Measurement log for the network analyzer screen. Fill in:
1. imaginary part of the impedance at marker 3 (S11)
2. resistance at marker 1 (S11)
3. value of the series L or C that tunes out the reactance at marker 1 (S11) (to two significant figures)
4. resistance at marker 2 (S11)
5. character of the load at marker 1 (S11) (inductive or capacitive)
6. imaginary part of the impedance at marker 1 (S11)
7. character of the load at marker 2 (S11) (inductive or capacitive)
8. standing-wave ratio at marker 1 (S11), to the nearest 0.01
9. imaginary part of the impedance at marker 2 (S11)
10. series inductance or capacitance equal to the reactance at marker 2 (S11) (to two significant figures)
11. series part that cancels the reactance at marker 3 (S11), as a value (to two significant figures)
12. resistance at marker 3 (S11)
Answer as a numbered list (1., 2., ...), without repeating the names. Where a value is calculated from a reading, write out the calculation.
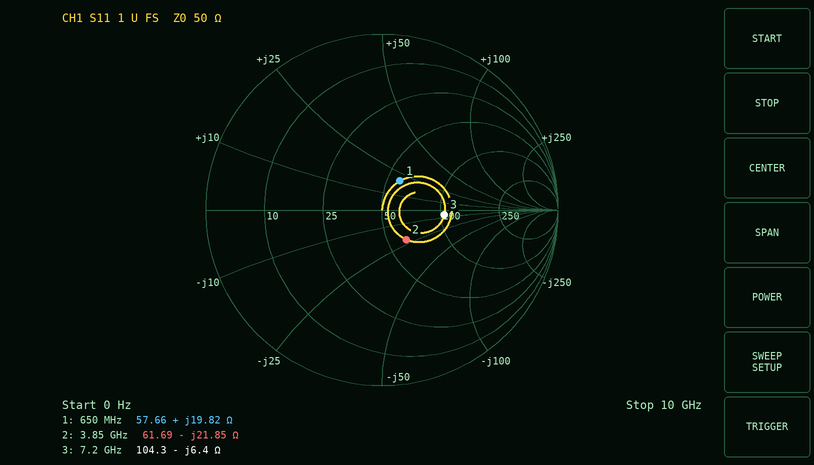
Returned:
1. -6.4 Ω
2. 57.66 Ω
3. C = 1/(2π × 650 MHz × 19.82 Ω) ≈ 12 pF
4. 61.69 Ω
5. inductive
6. +19.82 Ω
7. capacitive
8. 1.48
9. -21.85 Ω
10. C = 1/(2π × 3.85 GHz × 21.85 Ω) ≈ 1.9 pF
11. L = 6.4 Ω/(2π × 7.2 GHz) ≈ 141 pH, so 140 pH to two significant figures
12. 104.3 Ω
